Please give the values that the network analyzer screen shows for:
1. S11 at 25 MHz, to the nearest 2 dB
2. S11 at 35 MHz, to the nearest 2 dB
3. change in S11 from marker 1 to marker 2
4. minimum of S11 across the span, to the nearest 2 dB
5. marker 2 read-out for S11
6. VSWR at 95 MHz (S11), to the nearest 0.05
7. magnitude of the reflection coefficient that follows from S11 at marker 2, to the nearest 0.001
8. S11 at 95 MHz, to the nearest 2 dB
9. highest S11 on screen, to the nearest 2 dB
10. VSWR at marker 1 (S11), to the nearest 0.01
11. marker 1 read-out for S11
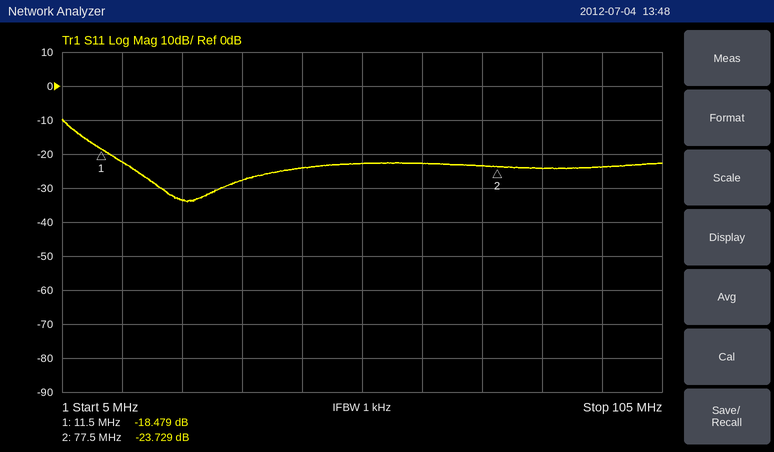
-34 dB
-28 dB
-5.250 dB
-34 dB
-23.729 dB
1.15
0.065
-24 dB
-10 dB
1.27
-18.479 dB
